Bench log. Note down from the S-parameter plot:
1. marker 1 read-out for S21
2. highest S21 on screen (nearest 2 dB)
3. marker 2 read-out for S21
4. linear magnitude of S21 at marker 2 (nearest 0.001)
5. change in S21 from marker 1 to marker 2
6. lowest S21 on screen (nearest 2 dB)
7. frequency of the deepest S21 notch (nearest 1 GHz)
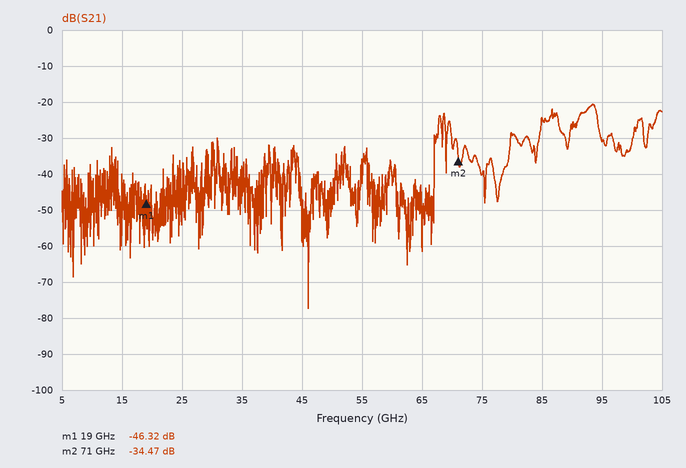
-46.32 dB
-20 dB
-34.47 dB
0.019
11.85 dB
-78 dB
46 GHz
